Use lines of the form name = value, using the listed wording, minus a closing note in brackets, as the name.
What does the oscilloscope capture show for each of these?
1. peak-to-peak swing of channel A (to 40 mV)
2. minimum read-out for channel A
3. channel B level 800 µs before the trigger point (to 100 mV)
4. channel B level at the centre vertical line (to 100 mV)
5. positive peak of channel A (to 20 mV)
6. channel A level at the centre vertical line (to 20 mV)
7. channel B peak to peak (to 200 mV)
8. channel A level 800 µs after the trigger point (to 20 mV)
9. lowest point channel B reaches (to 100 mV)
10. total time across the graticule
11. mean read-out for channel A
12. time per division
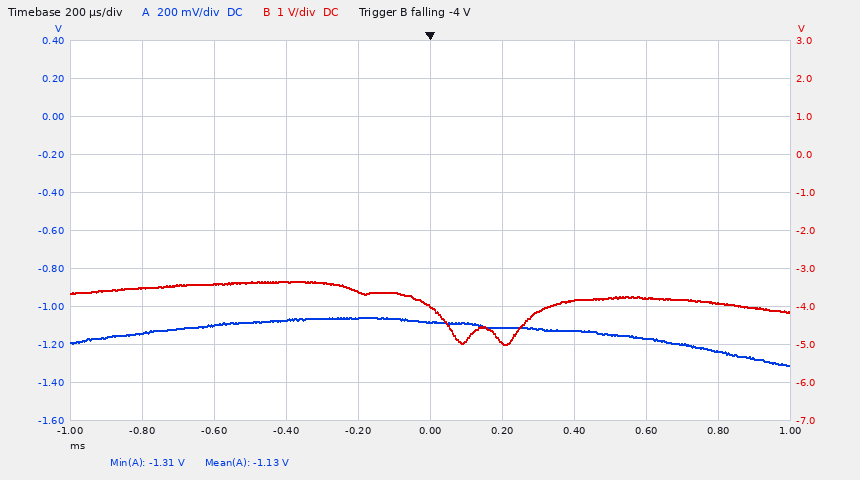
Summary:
peak-to-peak swing of channel A = 240 mV
minimum read-out for channel A = -1.31 V
channel B level 800 µs before the trigger point = -3.5 V
channel B level at the centre vertical line = -4.0 V
positive peak of channel A = -1.06 V
channel A level at the centre vertical line = -1.08 V
channel B peak to peak = 1.6 V
channel A level 800 µs after the trigger point = -1.24 V
lowest point channel B reaches = -5.0 V
total time across the graticule = 2 ms
mean read-out for channel A = -1.13 V
time per division = 200 µs
